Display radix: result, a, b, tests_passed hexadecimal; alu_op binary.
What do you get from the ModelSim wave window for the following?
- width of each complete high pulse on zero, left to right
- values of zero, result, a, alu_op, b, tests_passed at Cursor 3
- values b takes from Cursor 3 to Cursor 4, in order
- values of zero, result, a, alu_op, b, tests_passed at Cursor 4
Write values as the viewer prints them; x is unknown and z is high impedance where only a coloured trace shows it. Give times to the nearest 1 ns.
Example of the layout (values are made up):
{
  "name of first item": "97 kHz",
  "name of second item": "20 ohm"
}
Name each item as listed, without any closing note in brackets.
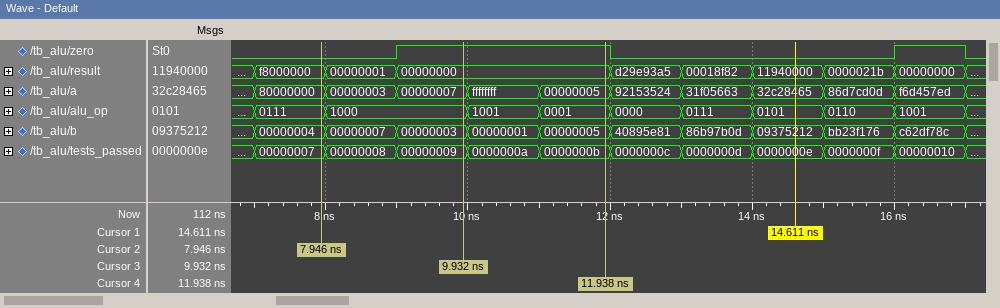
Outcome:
{
  "width of each complete high pulse on zero, left to right": "3 ns, 1 ns",
  "values of zero, result, a, alu_op, b, tests_passed at Cursor 3": "zero=1, result=00000000, a=00000007, alu_op=1000, b=00000003, tests_passed=00000009",
  "values b takes from Cursor 3 to Cursor 4, in order": "00000003, 00000001, 00000005",
  "values of zero, result, a, alu_op, b, tests_passed at Cursor 4": "zero=1, result=00000000, a=00000005, alu_op=0001, b=00000005, tests_passed=0000000b"
}
